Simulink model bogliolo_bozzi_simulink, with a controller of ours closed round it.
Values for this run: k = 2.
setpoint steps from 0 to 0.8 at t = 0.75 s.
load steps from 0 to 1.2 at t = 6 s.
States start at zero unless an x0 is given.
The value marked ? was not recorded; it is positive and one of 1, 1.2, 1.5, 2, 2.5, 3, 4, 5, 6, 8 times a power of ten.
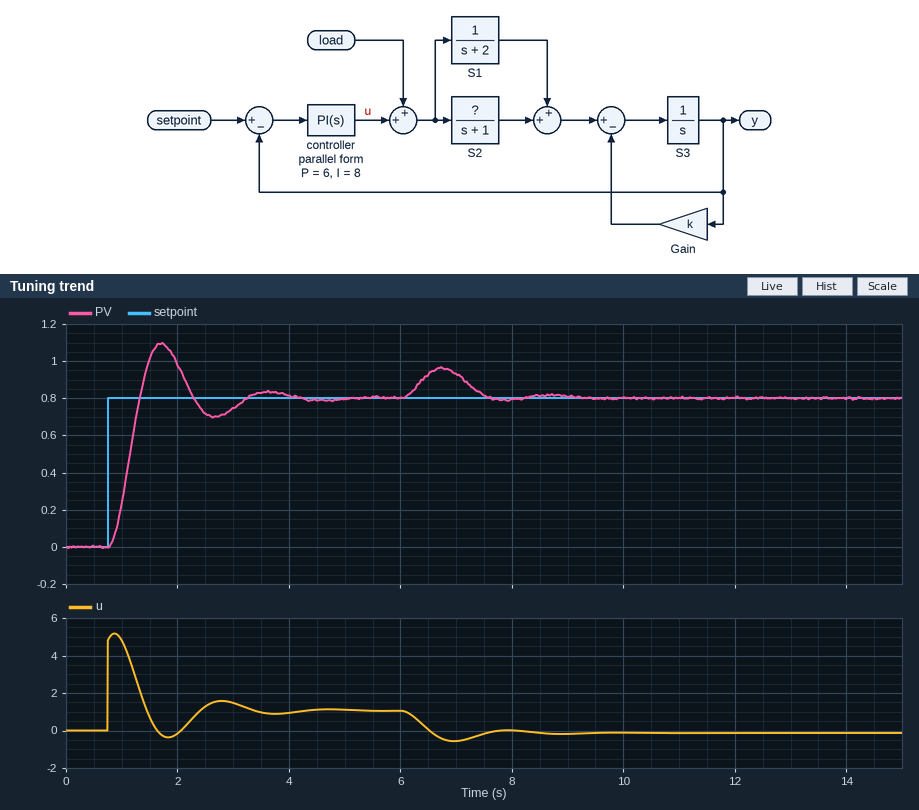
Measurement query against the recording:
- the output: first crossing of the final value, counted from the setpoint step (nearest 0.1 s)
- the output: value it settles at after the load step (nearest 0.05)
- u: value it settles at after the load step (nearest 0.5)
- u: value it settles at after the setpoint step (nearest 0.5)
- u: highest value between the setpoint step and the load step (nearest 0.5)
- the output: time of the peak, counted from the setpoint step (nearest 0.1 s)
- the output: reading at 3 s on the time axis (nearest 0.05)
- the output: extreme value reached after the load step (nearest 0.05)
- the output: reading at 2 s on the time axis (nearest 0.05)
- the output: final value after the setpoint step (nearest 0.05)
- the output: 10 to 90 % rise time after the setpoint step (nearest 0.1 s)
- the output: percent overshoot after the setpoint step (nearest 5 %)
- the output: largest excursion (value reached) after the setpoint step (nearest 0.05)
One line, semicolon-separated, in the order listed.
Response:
0.6 s; 0.80; 0.0; 1.0; 5.0; 1.0 s; 0.75; 0.95; 1.00; 0.80; 0.4 s; 35 %; 1.10
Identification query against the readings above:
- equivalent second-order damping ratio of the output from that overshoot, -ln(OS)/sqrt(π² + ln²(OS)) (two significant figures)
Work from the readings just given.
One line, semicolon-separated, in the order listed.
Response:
0.32
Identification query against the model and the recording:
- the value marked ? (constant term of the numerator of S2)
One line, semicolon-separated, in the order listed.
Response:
1
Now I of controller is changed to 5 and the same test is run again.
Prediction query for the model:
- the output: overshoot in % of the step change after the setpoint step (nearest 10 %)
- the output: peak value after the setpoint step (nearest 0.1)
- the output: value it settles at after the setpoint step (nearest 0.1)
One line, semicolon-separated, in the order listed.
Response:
20 %; 1.0; 0.8
